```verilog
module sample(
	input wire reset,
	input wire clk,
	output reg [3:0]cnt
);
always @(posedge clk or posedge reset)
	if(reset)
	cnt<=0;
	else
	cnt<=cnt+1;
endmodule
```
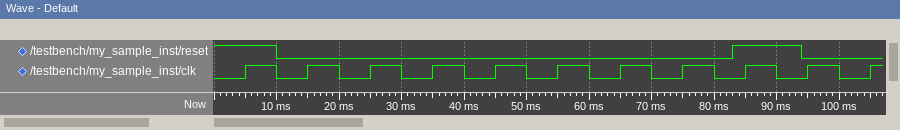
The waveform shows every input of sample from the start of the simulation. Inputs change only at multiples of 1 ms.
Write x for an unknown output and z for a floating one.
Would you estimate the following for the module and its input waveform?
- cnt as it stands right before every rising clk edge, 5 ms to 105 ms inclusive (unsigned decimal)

0, 0, 1, 2, 3, 4, 5, 6, 0, 0, 1
